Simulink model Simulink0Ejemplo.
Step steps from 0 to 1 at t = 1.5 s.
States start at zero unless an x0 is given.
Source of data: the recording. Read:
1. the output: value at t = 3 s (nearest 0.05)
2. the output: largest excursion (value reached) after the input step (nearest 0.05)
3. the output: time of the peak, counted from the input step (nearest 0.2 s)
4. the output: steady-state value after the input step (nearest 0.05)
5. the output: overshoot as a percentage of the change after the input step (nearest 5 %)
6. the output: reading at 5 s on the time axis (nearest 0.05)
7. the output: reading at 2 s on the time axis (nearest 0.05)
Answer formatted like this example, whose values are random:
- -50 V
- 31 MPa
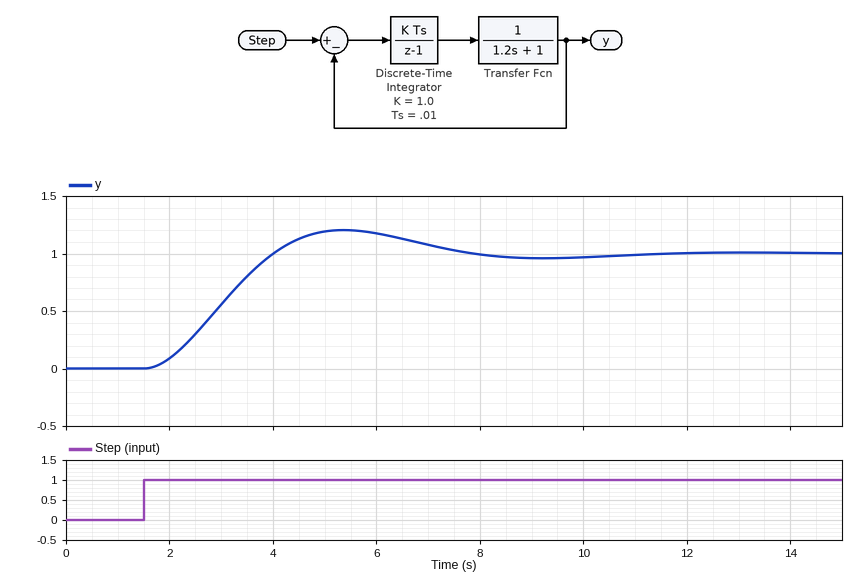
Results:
- 0.55
- 1.20
- 3.8 s
- 1.00
- 20 %
- 1.20
- 0.10
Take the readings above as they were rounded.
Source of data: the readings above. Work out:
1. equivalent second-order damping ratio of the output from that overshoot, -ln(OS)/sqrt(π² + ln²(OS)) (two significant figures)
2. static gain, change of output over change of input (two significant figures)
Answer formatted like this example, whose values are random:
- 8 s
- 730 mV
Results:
- 0.46
- 1.0
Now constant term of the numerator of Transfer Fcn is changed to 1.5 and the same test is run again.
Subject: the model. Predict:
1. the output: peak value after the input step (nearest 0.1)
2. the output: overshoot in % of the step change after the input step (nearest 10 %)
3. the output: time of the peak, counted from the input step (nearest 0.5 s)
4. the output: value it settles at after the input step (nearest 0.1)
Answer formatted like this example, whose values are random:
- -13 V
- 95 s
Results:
- 1.3
- 30 %
- 3.0 s
- 1.0
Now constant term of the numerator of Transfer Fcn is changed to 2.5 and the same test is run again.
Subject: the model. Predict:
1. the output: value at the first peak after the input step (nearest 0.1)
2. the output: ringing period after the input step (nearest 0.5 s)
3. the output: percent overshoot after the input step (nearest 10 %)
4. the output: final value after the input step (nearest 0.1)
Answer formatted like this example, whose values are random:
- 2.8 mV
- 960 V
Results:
- 1.4
- 4.5 s
- 40 %
- 1.0
